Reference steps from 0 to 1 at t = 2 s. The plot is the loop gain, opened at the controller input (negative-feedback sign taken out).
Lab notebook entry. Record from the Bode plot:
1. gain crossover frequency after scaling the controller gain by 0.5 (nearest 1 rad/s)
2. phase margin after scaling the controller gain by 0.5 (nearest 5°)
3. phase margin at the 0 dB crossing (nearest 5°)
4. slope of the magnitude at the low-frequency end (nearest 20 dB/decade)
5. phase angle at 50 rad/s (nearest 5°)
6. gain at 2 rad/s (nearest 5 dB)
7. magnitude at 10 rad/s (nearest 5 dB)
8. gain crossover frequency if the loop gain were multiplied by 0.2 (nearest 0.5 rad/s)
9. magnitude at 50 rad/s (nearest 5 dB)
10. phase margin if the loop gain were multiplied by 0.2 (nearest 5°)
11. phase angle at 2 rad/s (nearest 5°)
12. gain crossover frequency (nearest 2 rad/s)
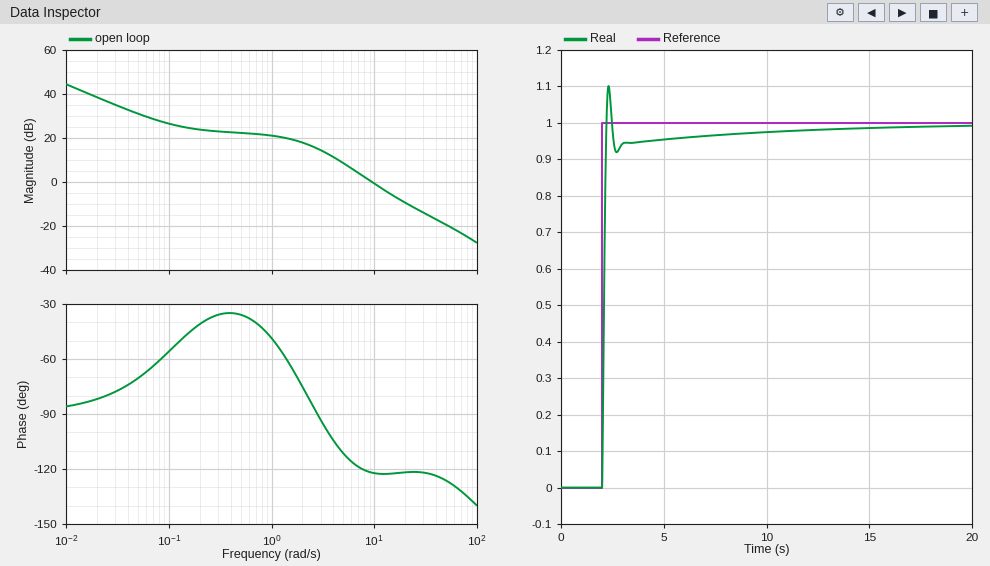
6 rad/s
65°
60°
-20 dB/decade
-125°
20 dB
0 dB
3.0 rad/s
-20 dB
85°
-75°
10 rad/s
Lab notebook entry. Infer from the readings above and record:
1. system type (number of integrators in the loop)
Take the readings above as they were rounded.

1
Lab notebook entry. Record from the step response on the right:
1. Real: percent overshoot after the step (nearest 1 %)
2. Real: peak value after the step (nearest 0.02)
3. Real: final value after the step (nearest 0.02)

10 %
1.10
1.00
